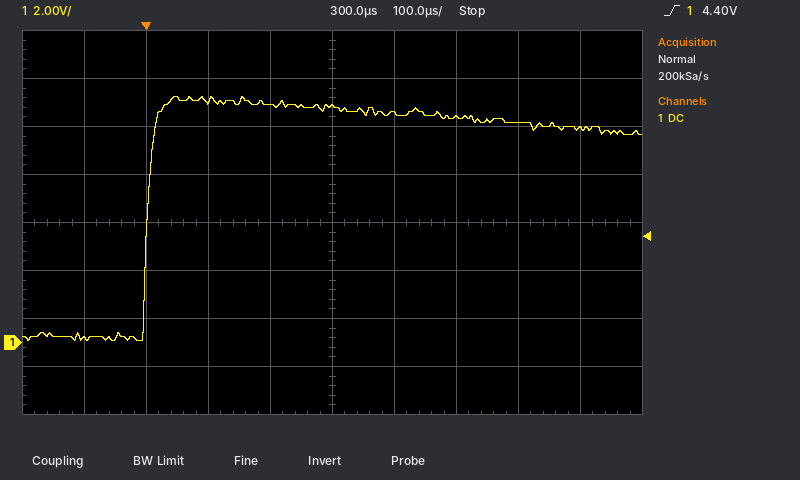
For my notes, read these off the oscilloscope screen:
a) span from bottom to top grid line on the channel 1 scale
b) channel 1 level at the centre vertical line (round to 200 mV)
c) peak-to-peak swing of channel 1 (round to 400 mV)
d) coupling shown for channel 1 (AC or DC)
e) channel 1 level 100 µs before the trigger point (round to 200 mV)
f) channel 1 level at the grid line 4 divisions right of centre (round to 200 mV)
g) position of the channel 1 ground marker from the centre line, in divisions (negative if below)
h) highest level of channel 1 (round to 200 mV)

16 V
9.8 V
10.0 V
DC
200 mV
9.0 V
-2.5 div
10.2 V
